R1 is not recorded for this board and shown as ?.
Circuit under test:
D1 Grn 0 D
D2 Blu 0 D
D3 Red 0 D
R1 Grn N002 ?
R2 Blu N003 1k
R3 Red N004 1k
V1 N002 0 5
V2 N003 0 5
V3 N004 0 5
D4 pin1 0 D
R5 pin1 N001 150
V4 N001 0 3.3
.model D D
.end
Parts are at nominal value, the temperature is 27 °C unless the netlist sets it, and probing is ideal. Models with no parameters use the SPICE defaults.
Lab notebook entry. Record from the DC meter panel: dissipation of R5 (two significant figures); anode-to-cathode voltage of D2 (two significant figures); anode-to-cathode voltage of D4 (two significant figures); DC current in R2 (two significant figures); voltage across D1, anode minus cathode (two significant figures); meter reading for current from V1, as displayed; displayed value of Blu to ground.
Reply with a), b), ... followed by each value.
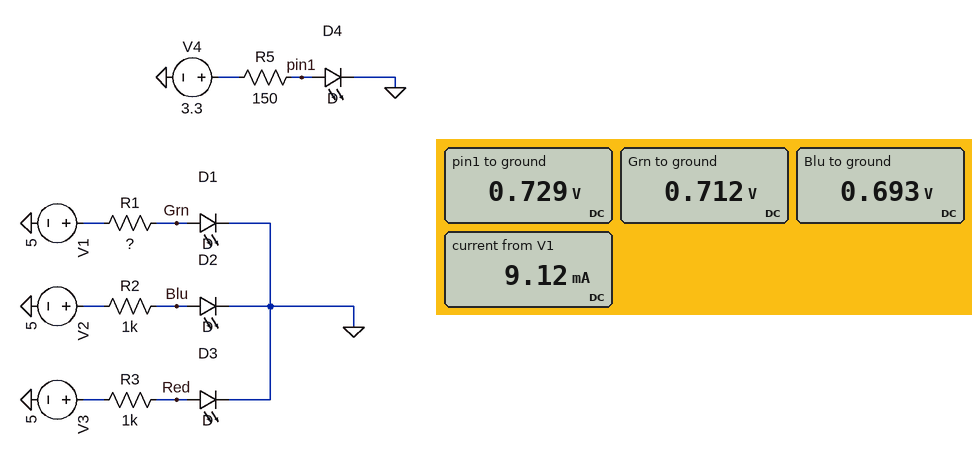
a) 44 mW
b) 690 mV
c) 730 mV
d) 4.3 mA
e) 710 mV
f) 9.12 mA
g) 0.693 V
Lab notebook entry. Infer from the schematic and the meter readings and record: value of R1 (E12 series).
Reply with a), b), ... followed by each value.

a) 470 Ω
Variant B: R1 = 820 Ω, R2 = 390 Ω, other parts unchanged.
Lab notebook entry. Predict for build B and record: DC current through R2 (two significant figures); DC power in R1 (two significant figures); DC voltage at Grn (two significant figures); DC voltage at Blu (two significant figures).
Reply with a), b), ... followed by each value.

a) 11 mA
b) 23 mW
c) 700 mV
d) 720 mV
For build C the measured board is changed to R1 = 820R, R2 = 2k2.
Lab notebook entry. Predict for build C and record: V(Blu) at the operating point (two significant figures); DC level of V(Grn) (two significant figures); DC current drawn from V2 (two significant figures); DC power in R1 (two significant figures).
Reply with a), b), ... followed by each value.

a) 670 mV
b) 700 mV
c) 2.0 mA
d) 23 mW
